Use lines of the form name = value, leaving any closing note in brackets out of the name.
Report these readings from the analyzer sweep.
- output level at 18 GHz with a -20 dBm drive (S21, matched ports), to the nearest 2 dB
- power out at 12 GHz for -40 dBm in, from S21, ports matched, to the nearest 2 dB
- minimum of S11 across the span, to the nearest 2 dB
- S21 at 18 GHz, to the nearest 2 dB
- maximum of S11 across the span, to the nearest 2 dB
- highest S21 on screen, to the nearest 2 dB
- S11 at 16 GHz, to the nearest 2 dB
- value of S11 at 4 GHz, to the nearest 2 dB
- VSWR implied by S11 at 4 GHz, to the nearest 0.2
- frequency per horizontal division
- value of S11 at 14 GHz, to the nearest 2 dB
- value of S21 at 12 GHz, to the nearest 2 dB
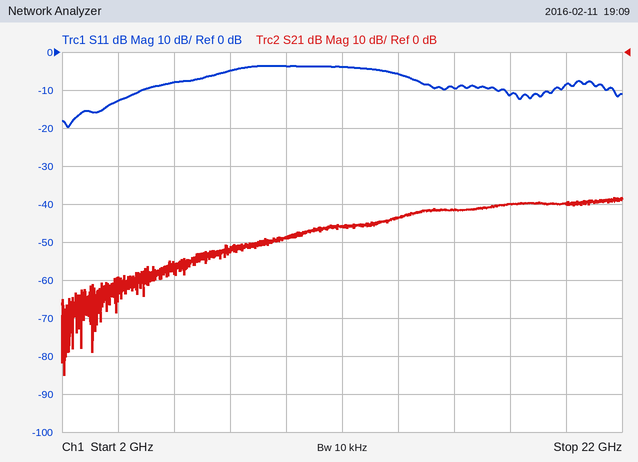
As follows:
output level at 18 GHz with a -20 dBm drive (S21, matched ports), to the nearest 2 dB = -60 dBm
power out at 12 GHz for -40 dBm in, from S21, ports matched, to the nearest 2 dB = -86 dBm
minimum of S11 across the span, to the nearest 2 dB = -20 dB
S21 at 18 GHz, to the nearest 2 dB = -40 dB
maximum of S11 across the span, to the nearest 2 dB = -4 dB
highest S21 on screen, to the nearest 2 dB = -38 dB
S11 at 16 GHz, to the nearest 2 dB = -10 dB
value of S11 at 4 GHz, to the nearest 2 dB = -12 dB
VSWR implied by S11 at 4 GHz, to the nearest 0.2 = 1.6
frequency per horizontal division = 2 GHz
value of S11 at 14 GHz, to the nearest 2 dB = -6 dB
value of S21 at 12 GHz, to the nearest 2 dB = -46 dB
